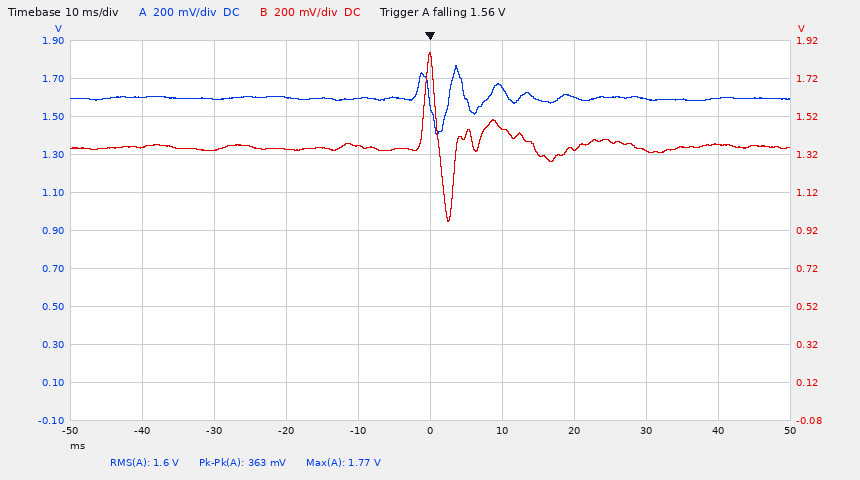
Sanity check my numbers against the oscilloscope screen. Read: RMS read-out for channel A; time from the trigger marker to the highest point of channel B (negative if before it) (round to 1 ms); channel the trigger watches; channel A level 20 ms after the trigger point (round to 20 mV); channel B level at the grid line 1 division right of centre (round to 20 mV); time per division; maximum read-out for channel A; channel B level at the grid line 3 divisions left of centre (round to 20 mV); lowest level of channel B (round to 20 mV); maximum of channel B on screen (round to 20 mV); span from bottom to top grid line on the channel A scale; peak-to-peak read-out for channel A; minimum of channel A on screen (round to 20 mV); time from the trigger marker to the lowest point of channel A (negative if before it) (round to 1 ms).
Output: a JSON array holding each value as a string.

["1.6 V", "0 ms", "channel A", "1.60 V", "1.46 V", "10 ms", "1.77 V", "1.34 V", "960 mV", "1.86 V", "2 V", "363 mV", "1.40 V", "+1 ms"]
